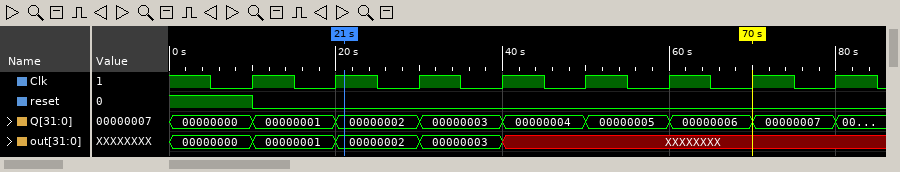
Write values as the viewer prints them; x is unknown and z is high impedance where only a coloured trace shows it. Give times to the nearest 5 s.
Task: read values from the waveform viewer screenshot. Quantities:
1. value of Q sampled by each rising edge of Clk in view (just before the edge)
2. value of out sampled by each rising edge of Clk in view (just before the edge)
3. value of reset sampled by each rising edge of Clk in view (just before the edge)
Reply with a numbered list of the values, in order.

1. 00000000, 00000001, 00000002, 00000003, 00000004, 00000005, 00000006, 00000007
2. 00000000, 00000001, 00000002, 00000003, XXXXXXXX, XXXXXXXX, XXXXXXXX, XXXXXXXX
3. 1 0 0 0 0 0 0 0
